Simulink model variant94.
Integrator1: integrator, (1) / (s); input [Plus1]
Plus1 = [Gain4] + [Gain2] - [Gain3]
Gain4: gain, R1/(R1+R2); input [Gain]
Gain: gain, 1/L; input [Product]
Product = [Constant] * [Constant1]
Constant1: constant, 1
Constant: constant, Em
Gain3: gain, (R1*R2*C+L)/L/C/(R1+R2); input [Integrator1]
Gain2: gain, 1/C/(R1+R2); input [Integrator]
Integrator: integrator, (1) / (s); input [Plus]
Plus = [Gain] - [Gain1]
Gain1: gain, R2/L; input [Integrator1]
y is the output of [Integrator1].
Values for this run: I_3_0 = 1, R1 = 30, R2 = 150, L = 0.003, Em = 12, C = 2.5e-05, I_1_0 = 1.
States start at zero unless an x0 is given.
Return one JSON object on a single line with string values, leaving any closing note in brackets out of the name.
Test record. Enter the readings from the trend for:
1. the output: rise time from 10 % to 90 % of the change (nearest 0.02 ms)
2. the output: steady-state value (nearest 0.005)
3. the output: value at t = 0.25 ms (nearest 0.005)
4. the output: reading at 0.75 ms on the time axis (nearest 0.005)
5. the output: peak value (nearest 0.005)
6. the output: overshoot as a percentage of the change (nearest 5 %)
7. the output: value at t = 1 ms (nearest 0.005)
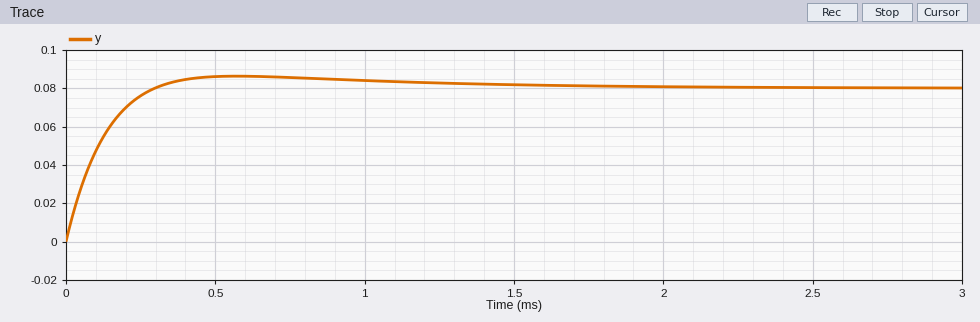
{"the output: rise time from 10 % to 90 % of the change": "0.20 ms", "the output: steady-state value": "0.080", "the output: value at t = 0.25 ms": "0.075", "the output: reading at 0.75 ms on the time axis": "0.085", "the output: peak value": "0.085", "the output: overshoot as a percentage of the change": "10 %", "the output: value at t = 1 ms": "0.085"}
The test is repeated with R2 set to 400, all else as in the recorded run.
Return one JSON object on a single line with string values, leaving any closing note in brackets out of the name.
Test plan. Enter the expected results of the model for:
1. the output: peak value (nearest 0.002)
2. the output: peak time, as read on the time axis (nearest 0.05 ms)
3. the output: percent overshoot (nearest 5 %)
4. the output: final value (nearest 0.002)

{"the output: peak value": "0.032", "the output: peak time, as read on the time axis": "0.50 ms", "the output: percent overshoot": "10 %", "the output: final value": "0.030"}
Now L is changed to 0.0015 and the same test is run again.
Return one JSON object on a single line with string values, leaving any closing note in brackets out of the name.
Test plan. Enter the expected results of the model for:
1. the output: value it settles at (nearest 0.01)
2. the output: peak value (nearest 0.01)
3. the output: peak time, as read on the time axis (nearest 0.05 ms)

{"the output: value it settles at": "0.08", "the output: peak value": "0.08", "the output: peak time, as read on the time axis": "0.35 ms"}
